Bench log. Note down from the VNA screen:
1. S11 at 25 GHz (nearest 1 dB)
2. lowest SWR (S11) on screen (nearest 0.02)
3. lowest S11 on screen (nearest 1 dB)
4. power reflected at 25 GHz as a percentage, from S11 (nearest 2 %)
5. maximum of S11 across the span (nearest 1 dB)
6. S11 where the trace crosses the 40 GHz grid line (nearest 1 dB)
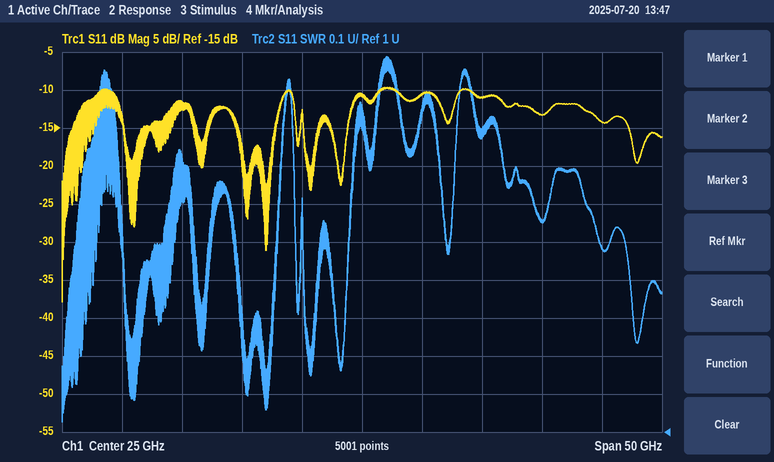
-11 dB
1.02
-38 dB
8 %
-10 dB
-13 dB
